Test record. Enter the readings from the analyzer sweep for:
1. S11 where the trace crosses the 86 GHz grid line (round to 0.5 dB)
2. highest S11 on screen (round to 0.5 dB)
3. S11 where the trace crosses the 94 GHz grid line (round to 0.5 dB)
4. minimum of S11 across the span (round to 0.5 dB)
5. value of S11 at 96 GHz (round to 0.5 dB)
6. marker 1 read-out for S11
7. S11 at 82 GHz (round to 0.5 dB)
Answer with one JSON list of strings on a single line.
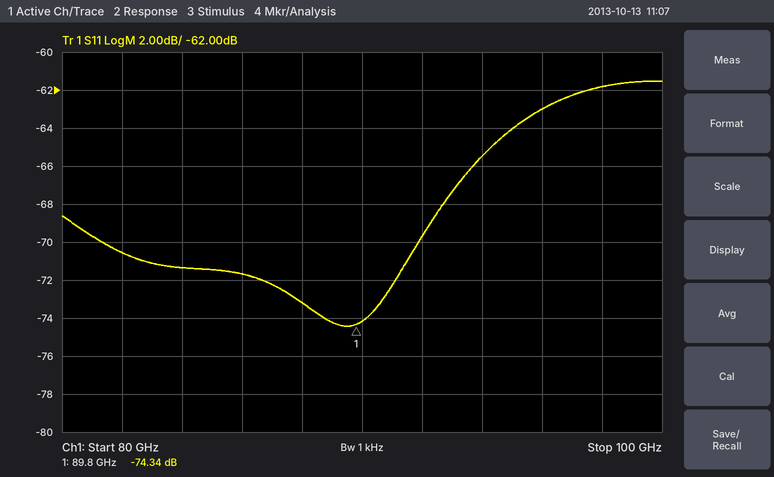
["-71.5 dB", "-61.5 dB", "-65.5 dB", "-74.5 dB", "-63.0 dB", "-74.34 dB", "-70.5 dB"]
